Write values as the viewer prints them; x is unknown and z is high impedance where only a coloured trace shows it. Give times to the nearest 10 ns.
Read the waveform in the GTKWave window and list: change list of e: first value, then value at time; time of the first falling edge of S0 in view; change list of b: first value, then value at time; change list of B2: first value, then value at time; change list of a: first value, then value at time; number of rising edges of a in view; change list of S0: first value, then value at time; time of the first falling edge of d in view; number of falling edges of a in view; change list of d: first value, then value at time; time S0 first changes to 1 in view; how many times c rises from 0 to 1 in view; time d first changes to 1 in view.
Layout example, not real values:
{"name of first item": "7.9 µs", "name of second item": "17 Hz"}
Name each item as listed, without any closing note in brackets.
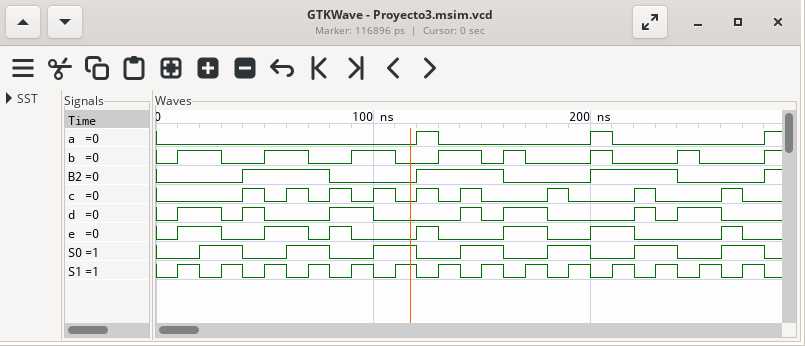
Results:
{"change list of e: first value, then value at time": "0, 1 at 10 ns, 0 at 30 ns, 1 at 50 ns, 0 at 70 ns, 1 at 80 ns, 0 at 90 ns, 1 at 120 ns, 0 at 130 ns, 1 at 160 ns, 0 at 180 ns, 1 at 200 ns, 0 at 220 ns, 1 at 260 ns, 0 at 270 ns", "time of the first falling edge of S0 in view": "40 ns", "change list of b: first value, then value at time": "0, 1 at 10 ns, 0 at 30 ns, 1 at 50 ns, 0 at 70 ns, 1 at 90 ns, 0 at 110 ns, 1 at 130 ns, 0 at 150 ns, 1 at 160 ns, 0 at 170 ns, 1 at 200 ns, 0 at 210 ns, 1 at 240 ns, 0 at 250 ns, 1 at 280 ns", "change list of B2: first value, then value at time": "0, 1 at 40 ns, 0 at 80 ns, 1 at 120 ns, 0 at 160 ns, 1 at 200 ns, 0 at 240 ns, 1 at 280 ns", "change list of a: first value, then value at time": "0, 1 at 120 ns, 0 at 130 ns, 1 at 200 ns, 0 at 210 ns, 1 at 280 ns", "number of rising edges of a in view": "3", "change list of S0: first value, then value at time": "0, 1 at 20 ns, 0 at 40 ns, 1 at 60 ns, 0 at 80 ns, 1 at 100 ns, 0 at 120 ns, 1 at 140 ns, 0 at 160 ns, 1 at 180 ns, 0 at 200 ns, 1 at 220 ns, 0 at 240 ns, 1 at 260 ns, 0 at 280 ns", "time of the first falling edge of d in view": "30 ns", "number of falling edges of a in view": "2", "change list of d: first value, then value at time": "0, 1 at 10 ns, 0 at 30 ns, 1 at 40 ns, 0 at 50 ns, 1 at 80 ns, 0 at 100 ns, 1 at 140 ns, 0 at 150 ns, 1 at 160 ns, 0 at 180 ns, 1 at 220 ns, 0 at 230 ns, 1 at 240 ns, 0 at 260 ns", "time S0 first changes to 1 in view": "20 ns", "how many times c rises from 0 to 1 in view": "9", "time d first changes to 1 in view": "10 ns"}
